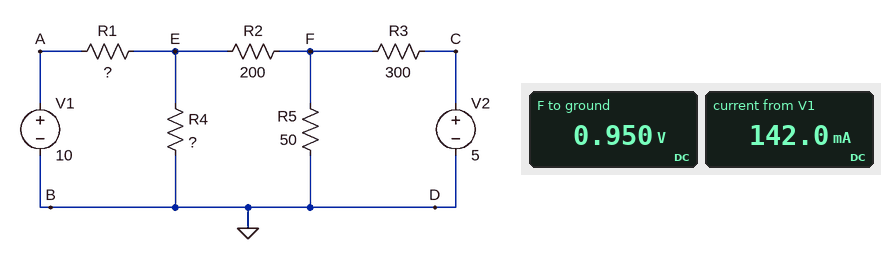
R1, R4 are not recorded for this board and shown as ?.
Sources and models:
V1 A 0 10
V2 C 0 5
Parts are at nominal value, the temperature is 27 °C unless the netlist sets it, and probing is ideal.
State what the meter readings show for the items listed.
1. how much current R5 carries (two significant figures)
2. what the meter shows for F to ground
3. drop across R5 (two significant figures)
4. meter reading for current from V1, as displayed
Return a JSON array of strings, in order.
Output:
["19 mA", "0.950 V", "950 mV", "142.0 mA"]
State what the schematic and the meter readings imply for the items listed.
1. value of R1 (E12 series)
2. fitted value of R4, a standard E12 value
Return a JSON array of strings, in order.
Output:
["56 Ω", "15 Ω"]
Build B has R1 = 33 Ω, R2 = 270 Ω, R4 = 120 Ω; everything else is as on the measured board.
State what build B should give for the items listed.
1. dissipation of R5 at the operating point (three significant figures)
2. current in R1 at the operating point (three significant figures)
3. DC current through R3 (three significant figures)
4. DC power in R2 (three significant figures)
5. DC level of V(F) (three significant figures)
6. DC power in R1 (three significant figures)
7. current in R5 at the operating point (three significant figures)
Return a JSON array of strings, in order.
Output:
["52.2 mW", "81.9 mA", "11.3 mA", "120 mW", "1.62 V", "221 mW", "32.3 mA"]
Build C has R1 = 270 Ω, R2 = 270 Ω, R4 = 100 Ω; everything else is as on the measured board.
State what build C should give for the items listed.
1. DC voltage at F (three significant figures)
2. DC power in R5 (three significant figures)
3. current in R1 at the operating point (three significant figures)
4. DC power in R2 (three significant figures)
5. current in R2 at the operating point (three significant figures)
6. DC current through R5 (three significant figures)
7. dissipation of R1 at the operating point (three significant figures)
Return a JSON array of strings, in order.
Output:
["935 mV", "17.5 mW", "28.4 mA", "7.17 mW", "5.15 mA", "18.7 mA", "218 mW"]
